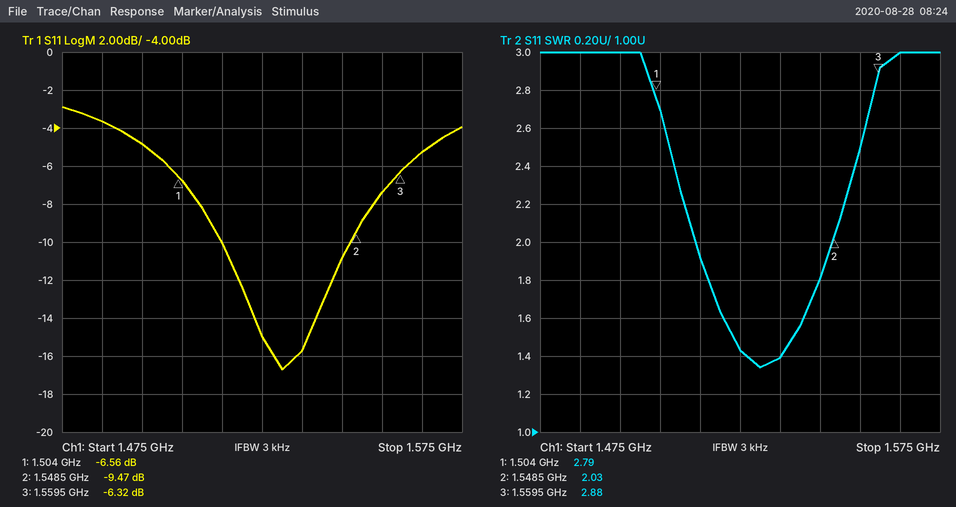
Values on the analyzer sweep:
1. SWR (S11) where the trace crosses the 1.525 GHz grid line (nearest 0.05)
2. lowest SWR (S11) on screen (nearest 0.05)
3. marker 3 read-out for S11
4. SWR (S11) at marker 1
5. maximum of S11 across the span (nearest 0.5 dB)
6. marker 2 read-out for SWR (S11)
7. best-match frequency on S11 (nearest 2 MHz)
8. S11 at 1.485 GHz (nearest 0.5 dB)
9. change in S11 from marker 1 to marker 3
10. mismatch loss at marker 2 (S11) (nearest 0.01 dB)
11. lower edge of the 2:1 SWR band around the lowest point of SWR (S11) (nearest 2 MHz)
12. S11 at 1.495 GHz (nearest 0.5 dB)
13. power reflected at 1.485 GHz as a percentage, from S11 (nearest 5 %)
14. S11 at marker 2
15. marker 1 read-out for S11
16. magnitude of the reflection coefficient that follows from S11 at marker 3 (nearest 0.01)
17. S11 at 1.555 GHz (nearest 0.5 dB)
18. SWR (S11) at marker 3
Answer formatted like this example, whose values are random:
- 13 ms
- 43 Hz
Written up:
- 1.45
- 1.35
- -6.32 dB
- 2.79
- -3.0 dB
- 2.03
- 1.530 GHz
- -3.5 dB
- 0.24 dB
- 0.52 dB
- 1.514 GHz
- -5.0 dB
- 45 %
- -9.47 dB
- -6.56 dB
- 0.48
- -7.5 dB
- 2.88
